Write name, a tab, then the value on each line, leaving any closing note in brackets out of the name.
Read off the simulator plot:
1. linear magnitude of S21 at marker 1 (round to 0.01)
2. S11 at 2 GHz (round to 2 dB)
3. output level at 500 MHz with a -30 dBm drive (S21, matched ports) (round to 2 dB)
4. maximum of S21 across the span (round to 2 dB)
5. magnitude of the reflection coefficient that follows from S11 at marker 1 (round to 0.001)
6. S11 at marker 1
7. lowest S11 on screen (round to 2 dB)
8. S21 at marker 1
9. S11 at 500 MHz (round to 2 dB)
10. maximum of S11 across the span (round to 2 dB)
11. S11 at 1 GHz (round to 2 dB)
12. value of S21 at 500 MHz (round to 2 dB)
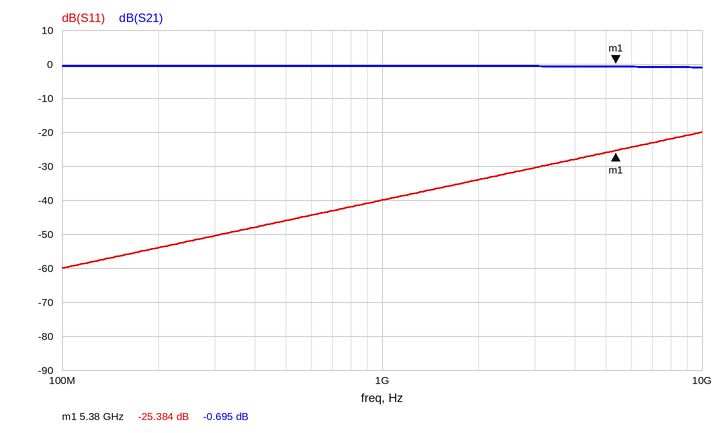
linear magnitude of S21 at marker 1	0.92
S11 at 2 GHz	-34 dB
output level at 500 MHz with a -30 dBm drive (S21, matched ports)	-30 dBm
maximum of S21 across the span	0 dB
magnitude of the reflection coefficient that follows from S11 at marker 1	0.054
S11 at marker 1	-25.384 dB
lowest S11 on screen	-60 dB
S21 at marker 1	-0.695 dB
S11 at 500 MHz	-46 dB
maximum of S11 across the span	-20 dB
S11 at 1 GHz	-40 dB
value of S21 at 500 MHz	0 dB
